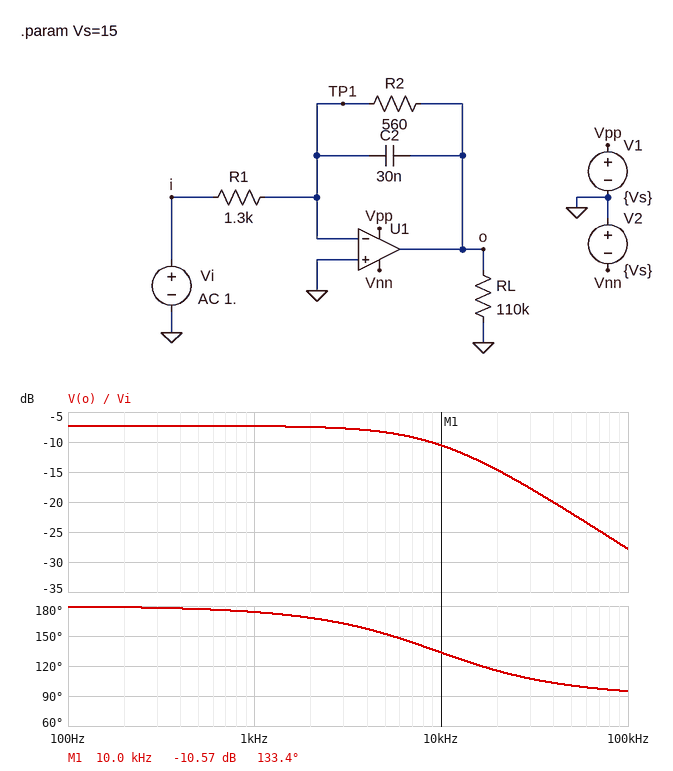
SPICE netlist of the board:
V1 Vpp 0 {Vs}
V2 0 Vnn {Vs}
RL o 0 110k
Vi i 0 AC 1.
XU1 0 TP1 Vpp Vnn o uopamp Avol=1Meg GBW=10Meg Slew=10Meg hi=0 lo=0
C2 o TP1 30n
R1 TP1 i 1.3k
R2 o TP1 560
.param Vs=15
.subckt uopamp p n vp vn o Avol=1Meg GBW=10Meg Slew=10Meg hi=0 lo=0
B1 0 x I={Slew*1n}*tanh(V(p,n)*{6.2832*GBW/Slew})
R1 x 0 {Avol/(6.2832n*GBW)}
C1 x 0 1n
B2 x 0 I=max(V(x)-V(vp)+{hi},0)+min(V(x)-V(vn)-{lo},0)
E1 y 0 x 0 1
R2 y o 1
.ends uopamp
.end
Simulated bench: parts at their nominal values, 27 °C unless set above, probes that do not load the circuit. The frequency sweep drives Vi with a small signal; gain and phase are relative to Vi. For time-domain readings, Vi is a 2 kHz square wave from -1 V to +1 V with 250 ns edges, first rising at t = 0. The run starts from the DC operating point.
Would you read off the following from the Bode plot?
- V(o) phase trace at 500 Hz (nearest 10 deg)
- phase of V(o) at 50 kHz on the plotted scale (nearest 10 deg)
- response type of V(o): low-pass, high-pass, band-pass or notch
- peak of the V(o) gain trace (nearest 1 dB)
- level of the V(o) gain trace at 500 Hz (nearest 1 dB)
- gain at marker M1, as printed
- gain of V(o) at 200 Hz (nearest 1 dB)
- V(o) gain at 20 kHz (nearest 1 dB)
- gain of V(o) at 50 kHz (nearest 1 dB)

180 deg
100 deg
low-pass
-7 dB
-7 dB
-10.57 dB
-7 dB
-15 dB
-22 dB
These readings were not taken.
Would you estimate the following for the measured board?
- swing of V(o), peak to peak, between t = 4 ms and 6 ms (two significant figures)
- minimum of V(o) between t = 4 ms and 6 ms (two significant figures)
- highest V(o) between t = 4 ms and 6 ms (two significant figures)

860 mV
-430 mV
430 mV
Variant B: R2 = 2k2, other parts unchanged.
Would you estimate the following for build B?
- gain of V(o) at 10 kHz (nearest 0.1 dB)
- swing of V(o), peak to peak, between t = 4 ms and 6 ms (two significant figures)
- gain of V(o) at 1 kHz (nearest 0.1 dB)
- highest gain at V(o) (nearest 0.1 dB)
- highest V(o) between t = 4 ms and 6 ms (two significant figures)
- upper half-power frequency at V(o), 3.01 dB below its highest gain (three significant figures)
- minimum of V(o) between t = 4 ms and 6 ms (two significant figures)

-8.0 dB
3.2 V
3.9 dB
4.6 dB
1.6 V
2.41 kHz
-1.6 V
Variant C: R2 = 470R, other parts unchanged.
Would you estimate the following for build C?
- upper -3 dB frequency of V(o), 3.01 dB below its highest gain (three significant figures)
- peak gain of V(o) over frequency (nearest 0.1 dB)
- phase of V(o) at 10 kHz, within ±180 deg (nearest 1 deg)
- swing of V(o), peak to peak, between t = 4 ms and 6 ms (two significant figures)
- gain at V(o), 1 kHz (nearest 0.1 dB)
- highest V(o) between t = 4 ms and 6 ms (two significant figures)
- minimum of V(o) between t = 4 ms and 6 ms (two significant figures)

11.3 kHz
-8.8 dB
138 deg
720 mV
-8.9 dB
360 mV
-360 mV
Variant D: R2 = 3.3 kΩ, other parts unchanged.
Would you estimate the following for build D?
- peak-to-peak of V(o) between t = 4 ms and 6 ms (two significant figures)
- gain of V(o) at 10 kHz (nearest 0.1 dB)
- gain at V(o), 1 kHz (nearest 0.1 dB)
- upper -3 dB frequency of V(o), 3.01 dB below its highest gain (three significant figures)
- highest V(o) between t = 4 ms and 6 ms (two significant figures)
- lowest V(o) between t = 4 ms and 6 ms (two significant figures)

4.3 V
-7.9 dB
6.7 dB
1.61 kHz
2.2 V
-2.2 V
